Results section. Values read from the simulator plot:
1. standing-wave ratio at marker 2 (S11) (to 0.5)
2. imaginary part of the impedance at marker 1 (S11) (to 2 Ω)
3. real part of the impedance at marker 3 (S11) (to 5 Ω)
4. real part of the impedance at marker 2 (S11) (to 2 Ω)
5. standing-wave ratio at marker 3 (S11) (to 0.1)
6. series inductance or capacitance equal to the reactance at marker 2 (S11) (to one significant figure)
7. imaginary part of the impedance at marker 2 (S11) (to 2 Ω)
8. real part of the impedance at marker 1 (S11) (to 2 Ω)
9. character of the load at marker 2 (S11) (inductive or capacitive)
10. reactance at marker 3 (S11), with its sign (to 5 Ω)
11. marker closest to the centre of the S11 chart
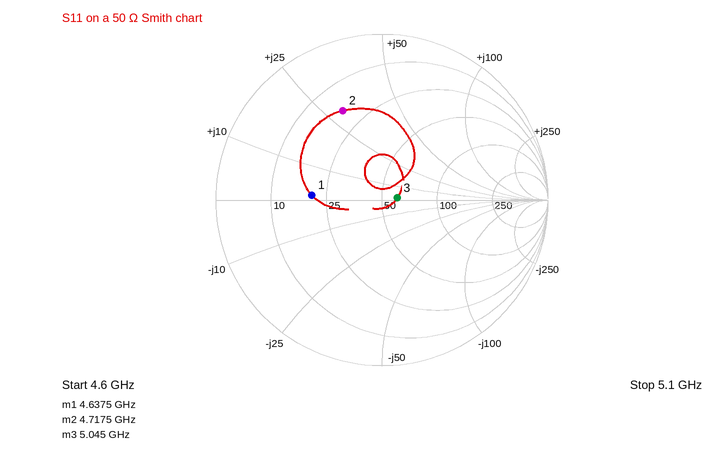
4.0
+2 Ω
60 Ω
18 Ω
1.2
1.0 nH
+30 Ω
20 Ω
inductive
0 Ω
marker 3
